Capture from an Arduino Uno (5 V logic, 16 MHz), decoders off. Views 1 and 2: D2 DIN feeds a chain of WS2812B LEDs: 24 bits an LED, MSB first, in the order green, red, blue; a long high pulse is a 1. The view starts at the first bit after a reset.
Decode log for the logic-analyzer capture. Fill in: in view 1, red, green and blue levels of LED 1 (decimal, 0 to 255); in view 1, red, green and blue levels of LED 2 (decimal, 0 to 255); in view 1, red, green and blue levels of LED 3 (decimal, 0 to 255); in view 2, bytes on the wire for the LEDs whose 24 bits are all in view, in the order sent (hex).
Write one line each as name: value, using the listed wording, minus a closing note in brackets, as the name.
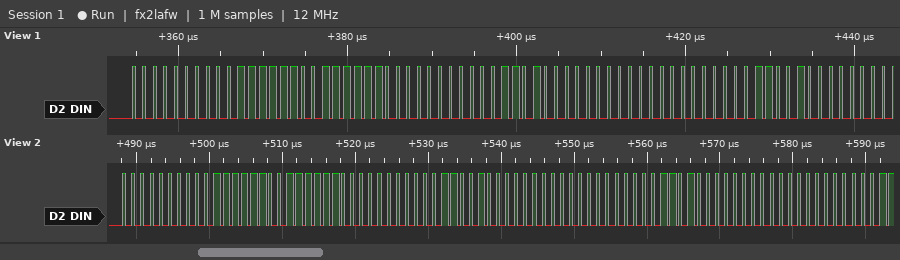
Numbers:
in view 1, red, green and blue levels of LED 1: 63, 0, 63
in view 1, red, green and blue levels of LED 2: 26, 0, 0
in view 1, red, green and blue levels of LED 3: 25, 0, 0
in view 2, bytes on the wire for the LEDs whose 24 bits are all in view, in the order sent: 00 3F 3F 00 19 00 00 1A 00
